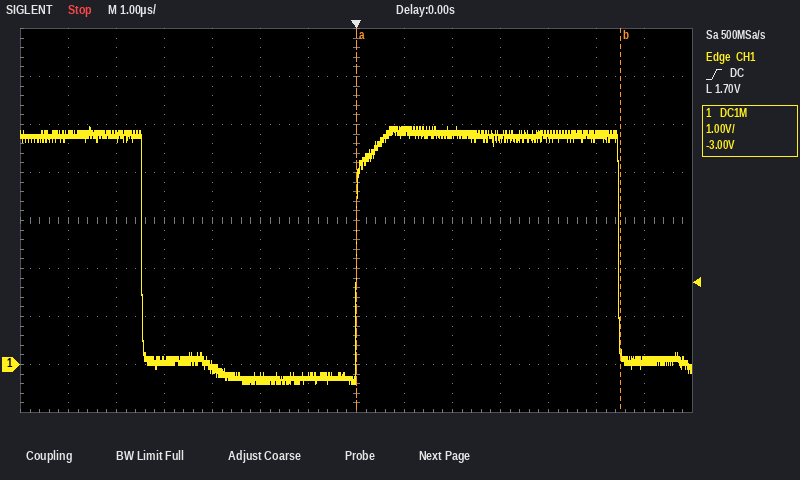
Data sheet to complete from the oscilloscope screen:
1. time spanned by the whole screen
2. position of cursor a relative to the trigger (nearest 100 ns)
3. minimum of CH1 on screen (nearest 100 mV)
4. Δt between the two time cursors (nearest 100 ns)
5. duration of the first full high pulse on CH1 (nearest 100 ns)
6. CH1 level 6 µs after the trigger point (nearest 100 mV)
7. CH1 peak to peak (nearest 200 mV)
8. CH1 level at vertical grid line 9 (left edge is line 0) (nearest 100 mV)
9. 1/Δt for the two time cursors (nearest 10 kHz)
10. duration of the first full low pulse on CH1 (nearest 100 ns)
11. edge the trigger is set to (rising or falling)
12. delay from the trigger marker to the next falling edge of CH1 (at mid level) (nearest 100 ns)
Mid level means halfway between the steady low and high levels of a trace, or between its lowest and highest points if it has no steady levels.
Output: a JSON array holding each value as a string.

["14 µs", "0.0 µs", "-400 mV", "5.5 µs", "5.5 µs", "100 mV", "5.4 V", "4.8 V", "180 kHz", "4.5 µs", "rising", "5.5 µs"]
